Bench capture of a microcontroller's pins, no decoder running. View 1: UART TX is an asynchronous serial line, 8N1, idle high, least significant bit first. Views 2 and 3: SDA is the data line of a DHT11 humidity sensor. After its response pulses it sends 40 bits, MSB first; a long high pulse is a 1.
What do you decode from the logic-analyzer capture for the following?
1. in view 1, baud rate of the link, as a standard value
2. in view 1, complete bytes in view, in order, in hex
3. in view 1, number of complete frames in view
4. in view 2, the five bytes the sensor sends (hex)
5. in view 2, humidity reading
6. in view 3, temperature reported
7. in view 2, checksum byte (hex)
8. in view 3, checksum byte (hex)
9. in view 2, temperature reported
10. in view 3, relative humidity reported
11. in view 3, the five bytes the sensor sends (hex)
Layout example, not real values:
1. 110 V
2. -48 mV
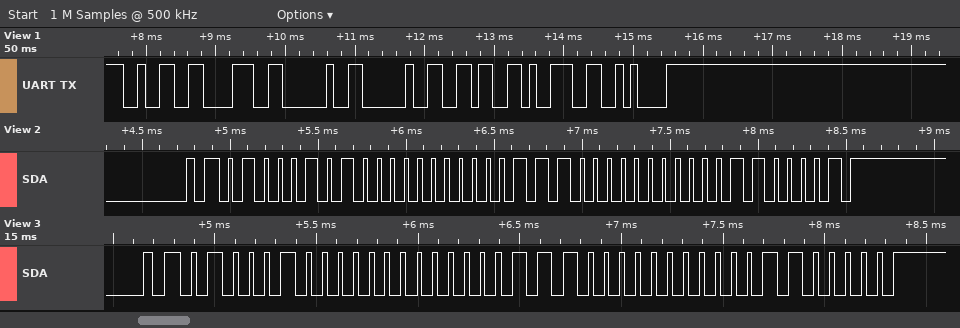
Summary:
1. 9600 baud
2. 32 38 20 20 36 39 0A
3. 7
4. 45 00 1C 00 61
5. 69 %
6. 28.0 °C
7. 0x61
8. 0x60
9. 28.0 °C
10. 68 %
11. 44 00 1C 00 60
